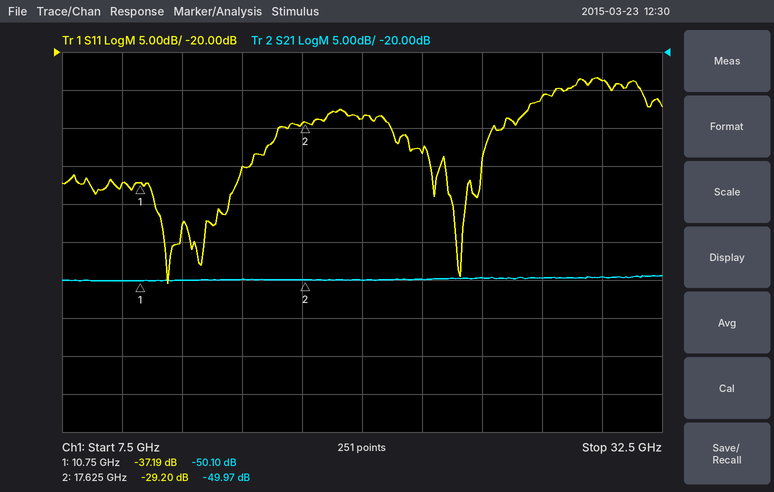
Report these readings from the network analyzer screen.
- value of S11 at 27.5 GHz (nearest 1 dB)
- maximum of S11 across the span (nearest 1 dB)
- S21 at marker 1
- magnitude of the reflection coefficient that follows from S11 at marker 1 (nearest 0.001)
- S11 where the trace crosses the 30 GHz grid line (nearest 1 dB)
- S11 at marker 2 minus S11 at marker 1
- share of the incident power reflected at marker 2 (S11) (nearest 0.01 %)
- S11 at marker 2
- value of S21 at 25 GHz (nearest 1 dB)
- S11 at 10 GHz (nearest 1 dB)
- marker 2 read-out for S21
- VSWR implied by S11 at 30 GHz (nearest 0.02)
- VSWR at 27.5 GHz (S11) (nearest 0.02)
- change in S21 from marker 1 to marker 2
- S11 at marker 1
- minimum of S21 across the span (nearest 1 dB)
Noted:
-26 dB
-23 dB
-50.10 dB
0.014
-24 dB
7.99 dB
0.12 %
-29.20 dB
-50 dB
-37 dB
-49.97 dB
1.14
1.10
0.13 dB
-37.19 dB
-50 dB
